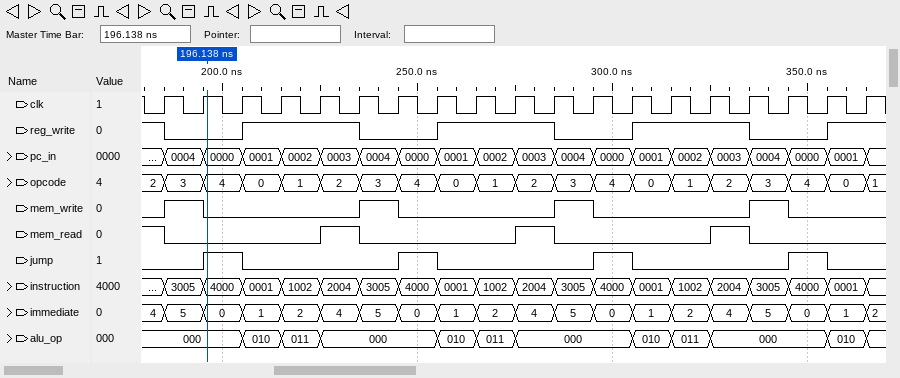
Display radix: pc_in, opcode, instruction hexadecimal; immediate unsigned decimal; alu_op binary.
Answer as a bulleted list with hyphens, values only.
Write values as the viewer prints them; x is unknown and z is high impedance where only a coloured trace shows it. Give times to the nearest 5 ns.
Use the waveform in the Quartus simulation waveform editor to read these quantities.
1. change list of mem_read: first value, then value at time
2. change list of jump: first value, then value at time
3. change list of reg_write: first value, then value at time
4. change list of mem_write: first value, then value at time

- 1, 0 at 185 ns, 1 at 225 ns, 0 at 235 ns, 1 at 275 ns, 0 at 285 ns, 1 at 325 ns, 0 at 335 ns
- 0, 1 at 195 ns, 0 at 205 ns, 1 at 245 ns, 0 at 255 ns, 1 at 295 ns, 0 at 305 ns, 1 at 345 ns, 0 at 355 ns
- 1, 0 at 185 ns, 1 at 205 ns, 0 at 235 ns, 1 at 255 ns, 0 at 285 ns, 1 at 305 ns, 0 at 335 ns, 1 at 355 ns
- 0, 1 at 185 ns, 0 at 195 ns, 1 at 235 ns, 0 at 245 ns, 1 at 285 ns, 0 at 295 ns, 1 at 335 ns, 0 at 345 ns
